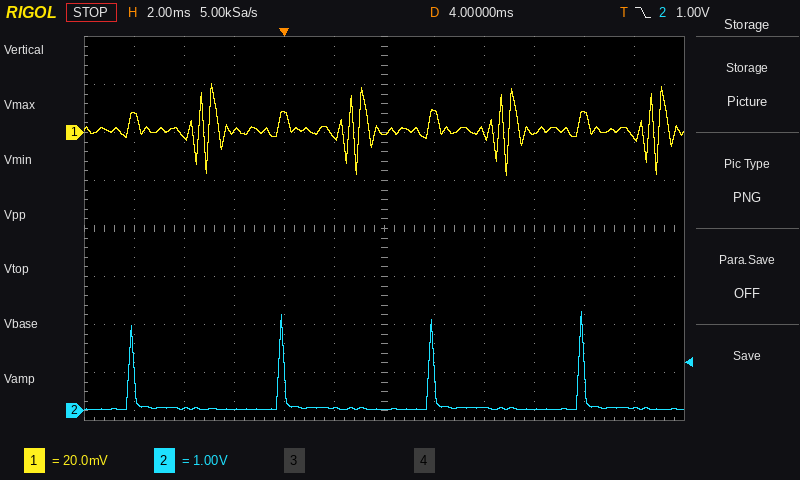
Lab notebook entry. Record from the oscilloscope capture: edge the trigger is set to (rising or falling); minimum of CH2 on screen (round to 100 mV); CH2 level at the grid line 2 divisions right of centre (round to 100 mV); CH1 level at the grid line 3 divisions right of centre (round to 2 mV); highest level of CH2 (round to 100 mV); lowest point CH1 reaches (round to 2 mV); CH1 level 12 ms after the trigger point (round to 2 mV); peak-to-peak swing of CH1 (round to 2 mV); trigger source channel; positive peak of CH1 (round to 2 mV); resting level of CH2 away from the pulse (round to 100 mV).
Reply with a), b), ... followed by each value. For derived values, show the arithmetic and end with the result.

a) falling
b) 0.0 V
c) 100 mV
d) 0 mV
e) 2.1 V
f) -18 mV
g) 8 mV
h) 20 mV − (-18 mV) = 38 mV
i) CH2
j) 20 mV
k) 0.0 V
